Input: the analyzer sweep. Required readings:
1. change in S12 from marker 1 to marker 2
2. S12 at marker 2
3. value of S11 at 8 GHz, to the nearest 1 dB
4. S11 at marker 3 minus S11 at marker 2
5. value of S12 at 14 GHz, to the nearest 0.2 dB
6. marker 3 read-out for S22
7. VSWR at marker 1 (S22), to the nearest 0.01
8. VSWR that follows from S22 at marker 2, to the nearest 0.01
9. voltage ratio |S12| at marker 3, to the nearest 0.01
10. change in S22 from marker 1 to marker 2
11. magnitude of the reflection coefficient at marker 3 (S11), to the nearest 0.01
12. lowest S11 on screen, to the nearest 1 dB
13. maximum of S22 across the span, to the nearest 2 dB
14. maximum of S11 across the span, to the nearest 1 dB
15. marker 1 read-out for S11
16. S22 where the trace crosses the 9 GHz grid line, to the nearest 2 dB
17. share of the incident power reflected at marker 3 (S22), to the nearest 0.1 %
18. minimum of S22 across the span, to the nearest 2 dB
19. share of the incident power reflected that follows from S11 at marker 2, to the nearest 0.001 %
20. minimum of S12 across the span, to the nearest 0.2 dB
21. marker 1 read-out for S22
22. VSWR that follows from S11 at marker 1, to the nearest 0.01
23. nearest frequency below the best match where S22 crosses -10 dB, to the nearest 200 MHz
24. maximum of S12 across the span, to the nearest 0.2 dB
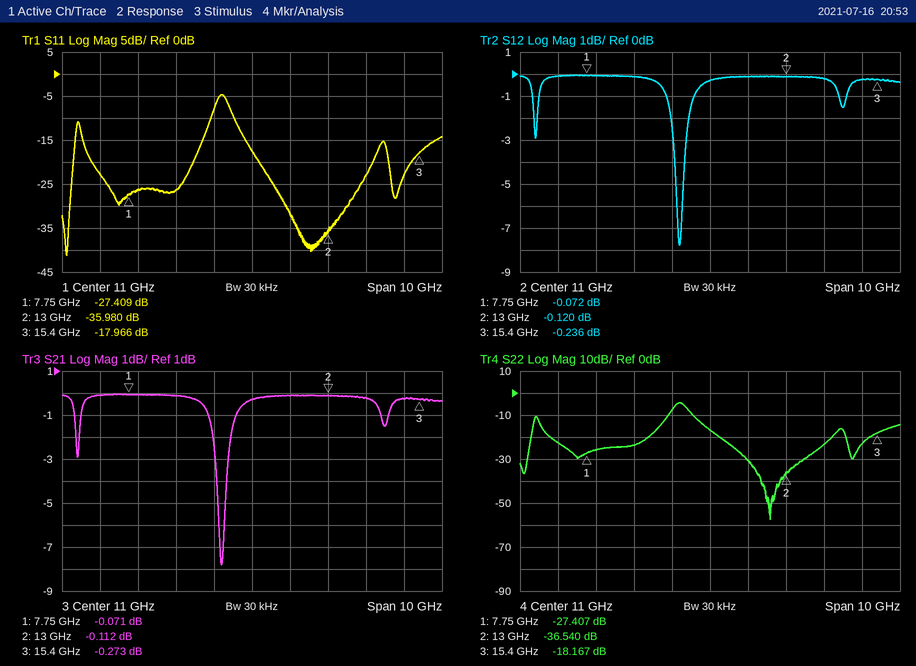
-0.048 dB
-0.120 dB
-26 dB
18.014 dB
-0.2 dB
-18.167 dB
1.09
1.03
0.97
-9.133 dB
0.13
-41 dB
-4 dB
-5 dB
-27.409 dB
-24 dB
1.5 %
-58 dB
0.025 %
-7.8 dB
-27.407 dB
1.09
10.6 GHz
0.0 dB
